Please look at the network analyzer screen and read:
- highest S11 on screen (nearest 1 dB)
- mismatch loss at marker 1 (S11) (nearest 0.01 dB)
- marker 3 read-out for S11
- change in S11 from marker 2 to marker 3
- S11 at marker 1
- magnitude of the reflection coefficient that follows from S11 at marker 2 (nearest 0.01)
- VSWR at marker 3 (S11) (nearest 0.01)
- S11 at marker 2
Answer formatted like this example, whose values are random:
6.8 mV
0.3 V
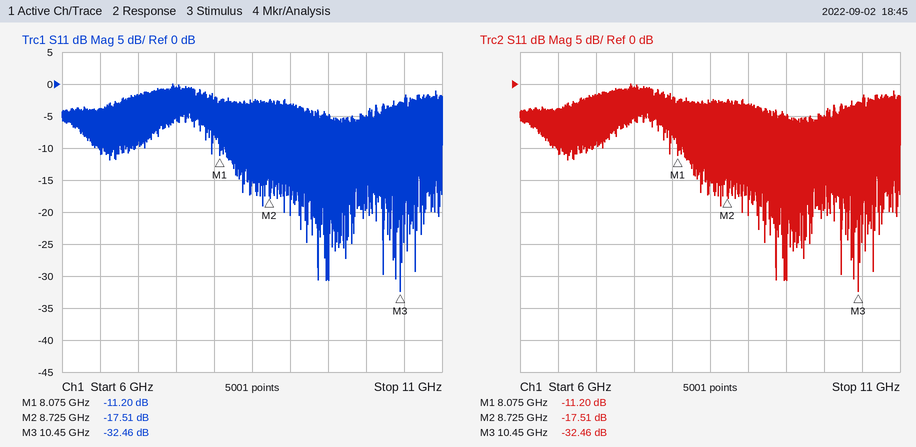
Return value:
0 dB
0.34 dB
-32.46 dB
-14.95 dB
-11.20 dB
0.13
1.05
-17.51 dB
